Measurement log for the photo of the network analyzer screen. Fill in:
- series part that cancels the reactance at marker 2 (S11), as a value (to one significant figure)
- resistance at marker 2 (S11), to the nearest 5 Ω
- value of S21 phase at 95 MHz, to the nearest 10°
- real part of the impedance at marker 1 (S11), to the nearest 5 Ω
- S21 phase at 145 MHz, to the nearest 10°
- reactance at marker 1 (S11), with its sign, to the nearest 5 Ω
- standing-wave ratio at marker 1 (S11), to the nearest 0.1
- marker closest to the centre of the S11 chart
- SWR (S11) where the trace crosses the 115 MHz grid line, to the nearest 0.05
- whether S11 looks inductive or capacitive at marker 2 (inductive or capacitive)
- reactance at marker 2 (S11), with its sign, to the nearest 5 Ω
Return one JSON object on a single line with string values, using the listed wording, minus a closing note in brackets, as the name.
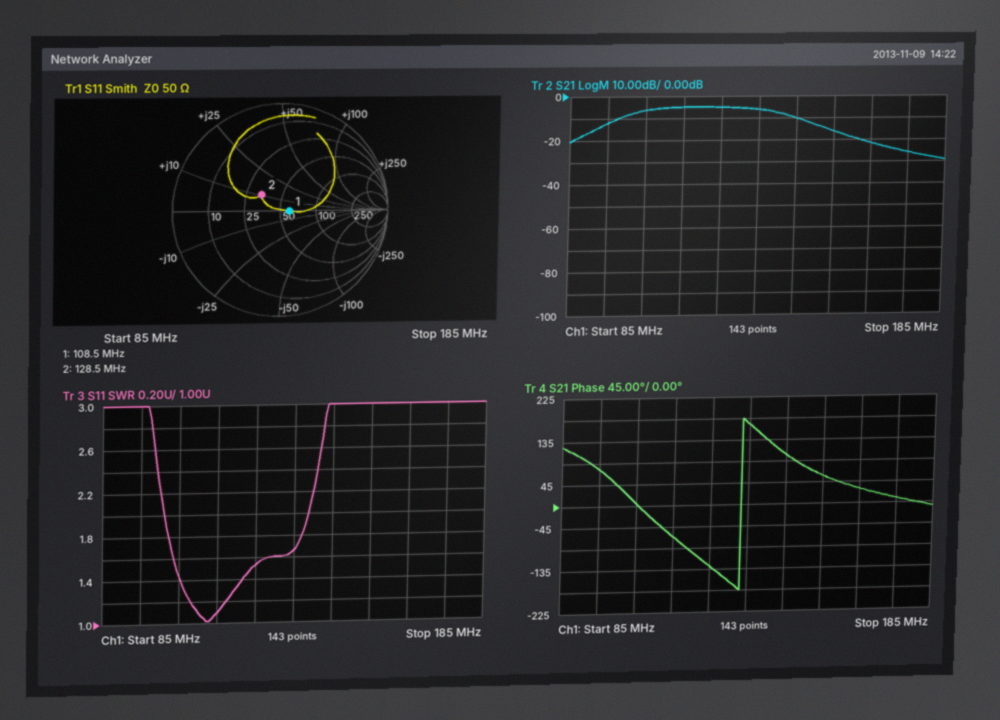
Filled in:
{"series part that cancels the reactance at marker 2 (S11), as a value": "100 pF", "resistance at marker 2 (S11), to the nearest 5 Ω": "35 Ω", "value of S21 phase at 95 MHz, to the nearest 10°": "80°", "real part of the impedance at marker 1 (S11), to the nearest 5 Ω": "60 Ω", "S21 phase at 145 MHz, to the nearest 10°": "100°", "reactance at marker 1 (S11), with its sign, to the nearest 5 Ω": "0 Ω", "standing-wave ratio at marker 1 (S11), to the nearest 0.1": "1.2", "marker closest to the centre of the S11 chart": "marker 1", "SWR (S11) where the trace crosses the 115 MHz grid line, to the nearest 0.05": "1.10", "whether S11 looks inductive or capacitive at marker 2": "inductive", "reactance at marker 2 (S11), with its sign, to the nearest 5 Ω": "+10 Ω"}
